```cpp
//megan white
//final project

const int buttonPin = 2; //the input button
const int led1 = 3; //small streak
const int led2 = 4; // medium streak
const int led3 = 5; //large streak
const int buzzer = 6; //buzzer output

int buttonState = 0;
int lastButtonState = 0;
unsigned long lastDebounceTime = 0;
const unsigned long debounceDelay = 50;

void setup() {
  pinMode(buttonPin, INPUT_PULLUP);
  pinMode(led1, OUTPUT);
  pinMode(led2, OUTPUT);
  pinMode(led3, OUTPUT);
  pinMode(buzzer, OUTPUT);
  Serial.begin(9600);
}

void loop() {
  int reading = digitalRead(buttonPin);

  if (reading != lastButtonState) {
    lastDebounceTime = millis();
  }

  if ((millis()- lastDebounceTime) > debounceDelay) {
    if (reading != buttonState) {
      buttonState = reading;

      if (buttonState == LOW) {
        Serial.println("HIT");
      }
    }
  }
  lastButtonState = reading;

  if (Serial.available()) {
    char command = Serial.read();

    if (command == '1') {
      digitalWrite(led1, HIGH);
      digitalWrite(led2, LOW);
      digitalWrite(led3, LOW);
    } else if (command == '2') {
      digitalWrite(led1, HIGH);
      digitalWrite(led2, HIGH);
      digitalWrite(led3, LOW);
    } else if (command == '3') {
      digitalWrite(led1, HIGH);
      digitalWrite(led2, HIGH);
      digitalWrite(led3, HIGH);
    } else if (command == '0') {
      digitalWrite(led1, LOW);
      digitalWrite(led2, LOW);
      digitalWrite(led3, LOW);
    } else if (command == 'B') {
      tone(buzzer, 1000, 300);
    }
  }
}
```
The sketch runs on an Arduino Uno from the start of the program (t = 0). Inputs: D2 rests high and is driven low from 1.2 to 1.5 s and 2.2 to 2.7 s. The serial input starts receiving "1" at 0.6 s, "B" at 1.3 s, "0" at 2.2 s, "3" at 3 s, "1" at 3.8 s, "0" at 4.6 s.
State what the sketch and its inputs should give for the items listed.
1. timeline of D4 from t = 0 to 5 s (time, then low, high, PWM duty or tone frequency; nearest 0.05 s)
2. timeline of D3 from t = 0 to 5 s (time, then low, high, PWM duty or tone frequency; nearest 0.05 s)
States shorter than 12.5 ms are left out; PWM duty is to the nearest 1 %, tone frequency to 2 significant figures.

0 s low; 3 s high; 3.8 s low
0 s low; 0.6 s high; 2.2 s low; 3 s high; 4.6 s low
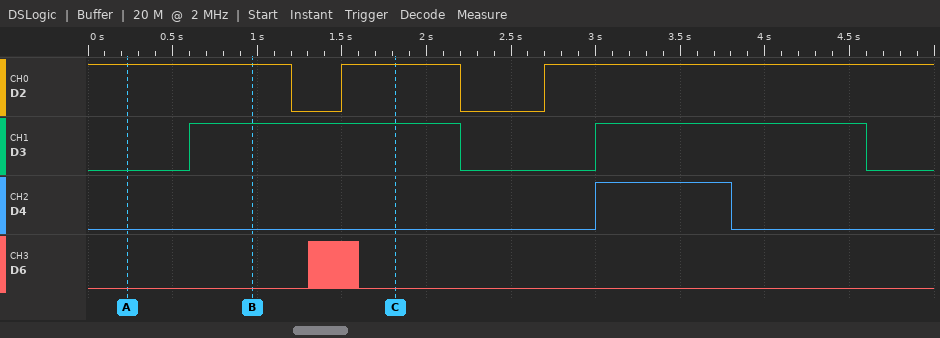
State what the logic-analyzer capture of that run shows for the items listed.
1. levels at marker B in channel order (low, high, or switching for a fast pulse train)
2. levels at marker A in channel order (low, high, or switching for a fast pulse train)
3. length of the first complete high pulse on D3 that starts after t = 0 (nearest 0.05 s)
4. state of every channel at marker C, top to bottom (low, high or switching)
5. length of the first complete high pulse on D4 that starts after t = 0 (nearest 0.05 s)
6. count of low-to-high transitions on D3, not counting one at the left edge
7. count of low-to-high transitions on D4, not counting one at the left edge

D2 high, D3 high, D4 low, D6 low
D2 high, D3 low, D4 low, D6 low
1.60 s
D2 high, D3 high, D4 low, D6 low
0.80 s
2
1
